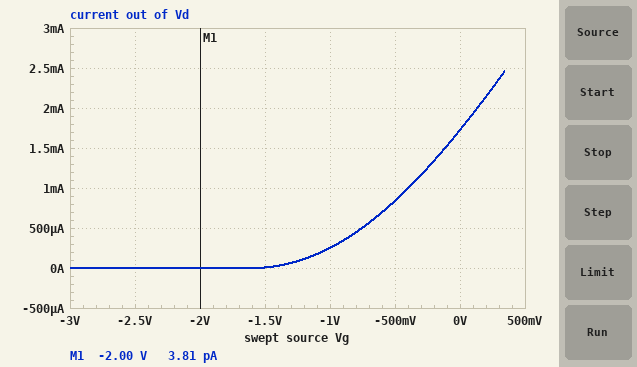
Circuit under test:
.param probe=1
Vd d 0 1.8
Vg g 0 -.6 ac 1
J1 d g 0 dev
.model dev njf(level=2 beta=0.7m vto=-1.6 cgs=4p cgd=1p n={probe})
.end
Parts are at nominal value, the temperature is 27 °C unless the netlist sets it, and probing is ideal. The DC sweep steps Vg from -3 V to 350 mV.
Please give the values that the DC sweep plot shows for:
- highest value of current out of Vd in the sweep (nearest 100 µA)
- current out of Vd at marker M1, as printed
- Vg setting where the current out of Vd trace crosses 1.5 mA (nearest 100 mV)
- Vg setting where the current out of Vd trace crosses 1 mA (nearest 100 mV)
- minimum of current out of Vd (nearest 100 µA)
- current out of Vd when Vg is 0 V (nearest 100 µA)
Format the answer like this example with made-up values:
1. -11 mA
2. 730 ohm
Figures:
1. 2.5 mA
2. 3.81 pA
3. -100 mV
4. -400 mV
5. 0 A
6. 1.7 mA
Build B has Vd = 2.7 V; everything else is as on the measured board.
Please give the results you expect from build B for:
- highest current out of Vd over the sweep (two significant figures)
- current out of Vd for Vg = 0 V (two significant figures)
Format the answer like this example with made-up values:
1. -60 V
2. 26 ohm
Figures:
1. 2.6 mA
2. 1.8 mA
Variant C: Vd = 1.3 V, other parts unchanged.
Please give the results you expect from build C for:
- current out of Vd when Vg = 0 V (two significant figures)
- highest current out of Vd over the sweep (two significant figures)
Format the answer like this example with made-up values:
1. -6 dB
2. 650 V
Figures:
1. 1.6 mA
2. 2.2 mA
